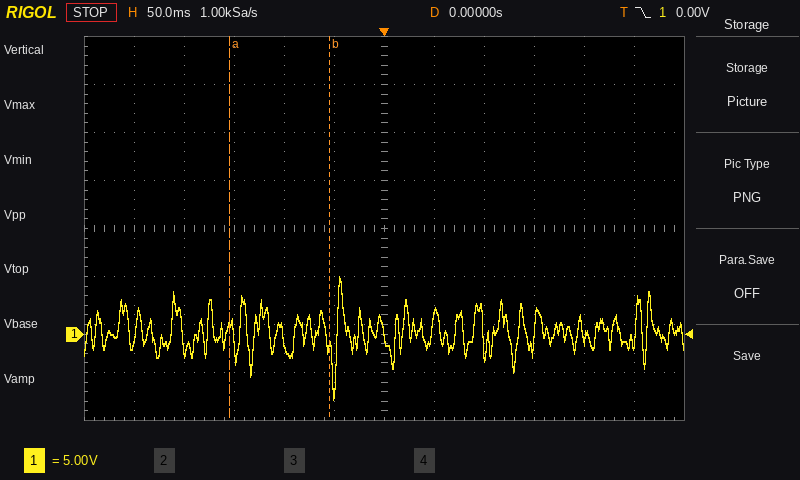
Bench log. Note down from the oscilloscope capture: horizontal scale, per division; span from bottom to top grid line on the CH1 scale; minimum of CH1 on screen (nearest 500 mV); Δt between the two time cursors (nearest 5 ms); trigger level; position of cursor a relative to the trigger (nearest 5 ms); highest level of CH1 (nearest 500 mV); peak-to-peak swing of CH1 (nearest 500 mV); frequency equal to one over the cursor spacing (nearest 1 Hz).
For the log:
50 ms
40 V
-7.0 V
100 ms
0.00 V
-155 ms
6.0 V
13.0 V
10 Hz
